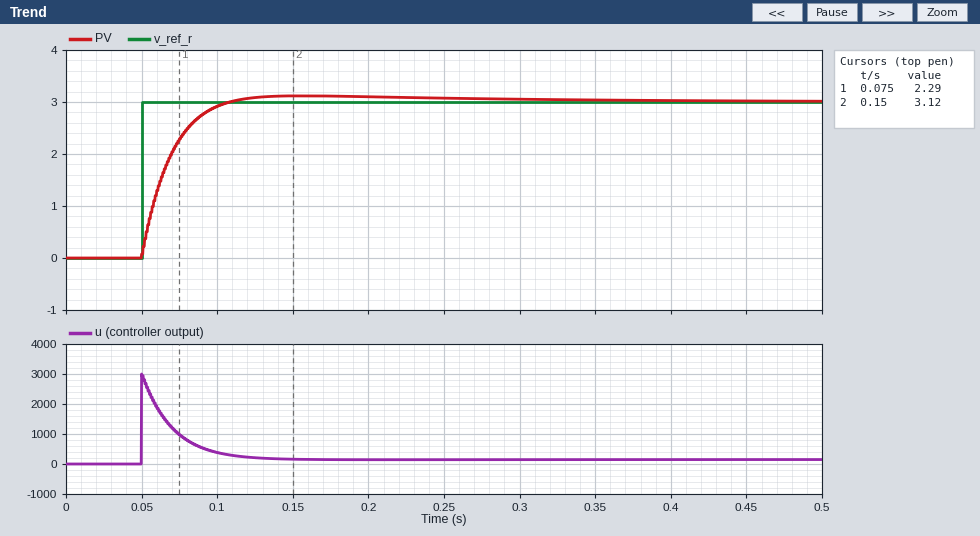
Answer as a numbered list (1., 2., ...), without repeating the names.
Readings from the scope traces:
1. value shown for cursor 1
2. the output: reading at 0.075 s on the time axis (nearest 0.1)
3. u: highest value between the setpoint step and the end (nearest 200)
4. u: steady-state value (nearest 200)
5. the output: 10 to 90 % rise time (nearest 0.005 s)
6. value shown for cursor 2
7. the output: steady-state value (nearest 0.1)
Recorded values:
1. 2.29
2. 2.3
3. 3000
4. 200
5. 0.035 s
6. 3.12
7. 3.0
